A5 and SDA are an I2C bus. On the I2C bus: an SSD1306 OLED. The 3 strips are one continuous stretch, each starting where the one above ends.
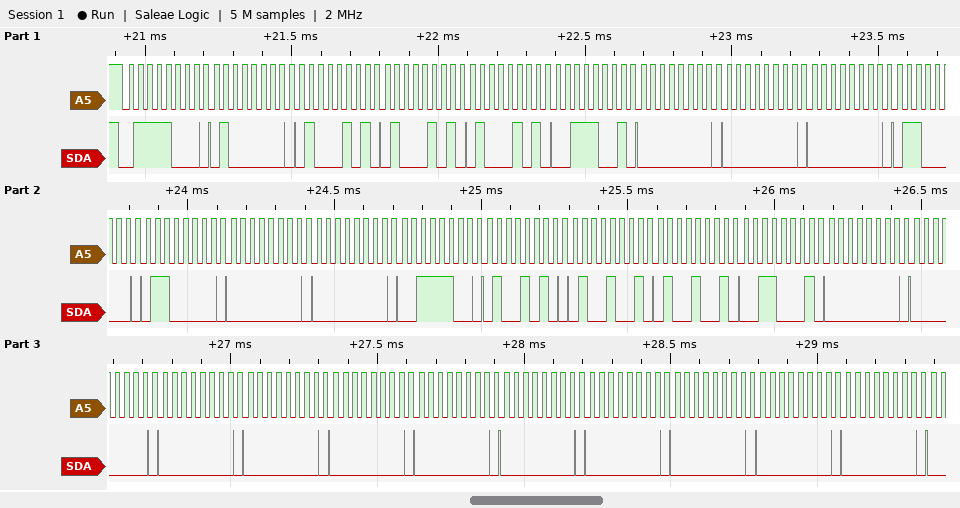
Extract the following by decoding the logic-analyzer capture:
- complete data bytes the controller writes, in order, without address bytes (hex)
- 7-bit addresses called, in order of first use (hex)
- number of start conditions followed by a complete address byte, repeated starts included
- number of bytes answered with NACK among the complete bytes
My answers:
40 45 45 45 39 00 00 00 60 60 00 00 3C 4A 49 49 31 00 00 00 00 00 00 00 00 00 00 00
0x3C
1
0
